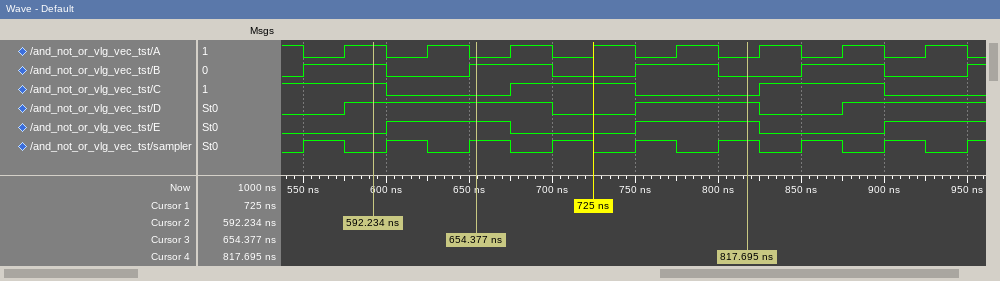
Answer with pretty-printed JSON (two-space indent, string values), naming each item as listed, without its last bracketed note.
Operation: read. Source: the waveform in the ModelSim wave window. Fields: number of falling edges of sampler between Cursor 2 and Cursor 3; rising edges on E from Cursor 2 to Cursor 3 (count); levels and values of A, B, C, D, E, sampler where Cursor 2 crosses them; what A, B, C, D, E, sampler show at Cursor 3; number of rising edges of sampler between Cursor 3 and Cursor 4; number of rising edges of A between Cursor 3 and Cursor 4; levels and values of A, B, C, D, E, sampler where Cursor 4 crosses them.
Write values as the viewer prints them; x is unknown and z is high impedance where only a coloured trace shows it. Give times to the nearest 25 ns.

{
  "number of falling edges of sampler between Cursor 2 and Cursor 3": "1",
  "rising edges on E from Cursor 2 to Cursor 3": "1",
  "levels and values of A, B, C, D, E, sampler where Cursor 2 crosses them": "A=1, B=1, C=1, D=1, E=0, sampler=0",
  "what A, B, C, D, E, sampler show at Cursor 3": "A=0, B=1, C=0, D=1, E=1, sampler=1",
  "number of rising edges of sampler between Cursor 3 and Cursor 4": "3",
  "number of rising edges of A between Cursor 3 and Cursor 4": "3",
  "levels and values of A, B, C, D, E, sampler where Cursor 4 crosses them": "A=0, B=0, C=0, D=1, E=1, sampler=1"
}
